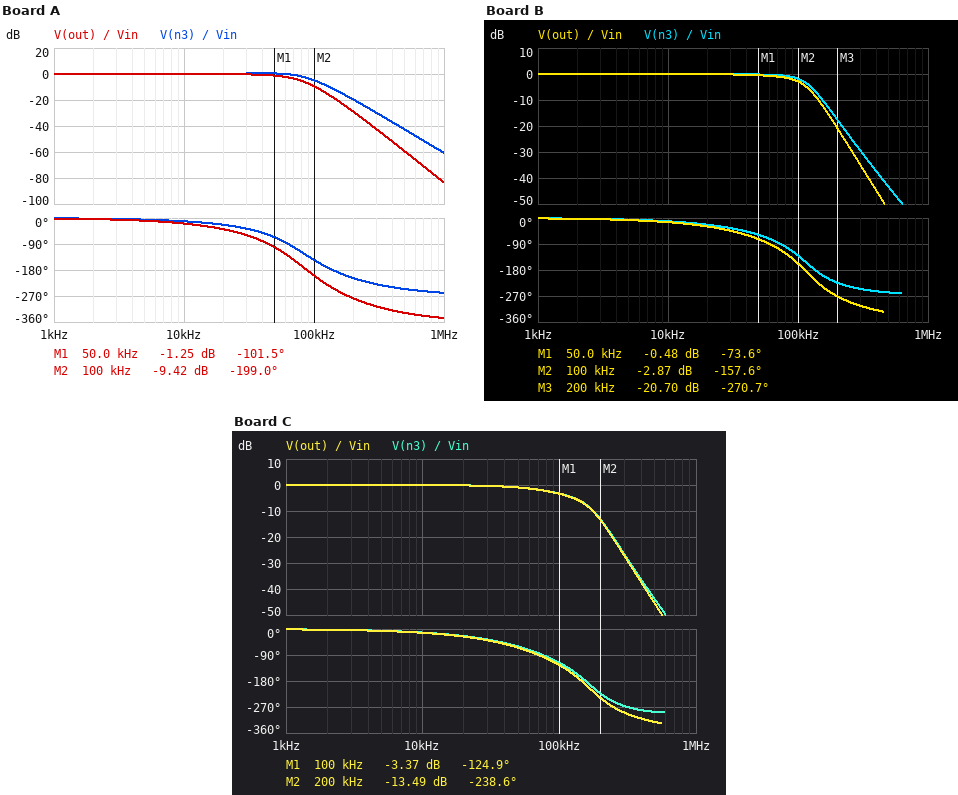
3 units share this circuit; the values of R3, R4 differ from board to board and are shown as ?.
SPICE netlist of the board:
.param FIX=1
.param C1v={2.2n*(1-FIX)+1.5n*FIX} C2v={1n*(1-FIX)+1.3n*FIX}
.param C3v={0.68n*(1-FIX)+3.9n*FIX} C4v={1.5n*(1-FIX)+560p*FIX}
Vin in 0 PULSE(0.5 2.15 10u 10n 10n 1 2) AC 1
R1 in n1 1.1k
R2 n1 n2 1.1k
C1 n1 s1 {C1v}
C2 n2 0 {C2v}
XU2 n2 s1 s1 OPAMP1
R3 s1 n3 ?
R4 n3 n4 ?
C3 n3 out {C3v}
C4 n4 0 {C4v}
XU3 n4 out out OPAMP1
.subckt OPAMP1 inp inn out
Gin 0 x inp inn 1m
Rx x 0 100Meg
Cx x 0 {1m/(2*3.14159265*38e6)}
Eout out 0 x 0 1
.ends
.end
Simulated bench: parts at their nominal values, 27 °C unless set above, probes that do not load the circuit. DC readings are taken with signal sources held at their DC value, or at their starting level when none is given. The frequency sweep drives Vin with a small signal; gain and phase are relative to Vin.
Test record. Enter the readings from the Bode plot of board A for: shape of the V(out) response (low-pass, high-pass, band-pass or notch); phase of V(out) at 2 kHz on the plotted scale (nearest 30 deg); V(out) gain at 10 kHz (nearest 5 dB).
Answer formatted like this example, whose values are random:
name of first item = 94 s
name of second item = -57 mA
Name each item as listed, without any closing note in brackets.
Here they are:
shape of the V(out) response = low-pass
phase of V(out) at 2 kHz on the plotted scale = 0 deg
V(out) gain at 10 kHz = 0 dB
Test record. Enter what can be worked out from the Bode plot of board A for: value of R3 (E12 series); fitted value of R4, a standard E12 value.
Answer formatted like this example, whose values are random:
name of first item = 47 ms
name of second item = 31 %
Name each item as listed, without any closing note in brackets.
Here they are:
value of R3 = 470 Ω
fitted value of R4, a standard E12 value = 3.9 kΩ
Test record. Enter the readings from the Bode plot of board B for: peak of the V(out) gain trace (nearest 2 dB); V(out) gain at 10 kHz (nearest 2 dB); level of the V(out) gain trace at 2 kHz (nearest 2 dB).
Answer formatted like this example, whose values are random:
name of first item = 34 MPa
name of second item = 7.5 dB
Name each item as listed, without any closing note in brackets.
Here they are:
peak of the V(out) gain trace = 0 dB
V(out) gain at 10 kHz = 0 dB
level of the V(out) gain trace at 2 kHz = 0 dB
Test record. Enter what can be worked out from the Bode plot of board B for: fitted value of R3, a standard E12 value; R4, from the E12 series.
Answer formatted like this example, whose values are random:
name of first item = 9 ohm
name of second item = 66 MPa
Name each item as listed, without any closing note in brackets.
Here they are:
fitted value of R3, a standard E12 value = 560 Ω
R4, from the E12 series = 1.5 kΩ
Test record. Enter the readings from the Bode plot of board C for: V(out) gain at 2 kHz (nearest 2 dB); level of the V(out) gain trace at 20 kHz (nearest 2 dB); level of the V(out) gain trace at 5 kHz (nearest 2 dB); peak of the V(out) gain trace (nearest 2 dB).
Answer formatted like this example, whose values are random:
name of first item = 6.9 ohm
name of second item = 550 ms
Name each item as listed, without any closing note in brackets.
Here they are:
V(out) gain at 2 kHz = 0 dB
level of the V(out) gain trace at 20 kHz = 0 dB
level of the V(out) gain trace at 5 kHz = 0 dB
peak of the V(out) gain trace = 0 dB
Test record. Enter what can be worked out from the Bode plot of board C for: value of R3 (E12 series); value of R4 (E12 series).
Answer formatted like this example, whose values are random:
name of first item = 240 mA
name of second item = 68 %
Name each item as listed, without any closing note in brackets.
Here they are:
value of R3 = 1 kΩ
value of R4 = 390 Ω
